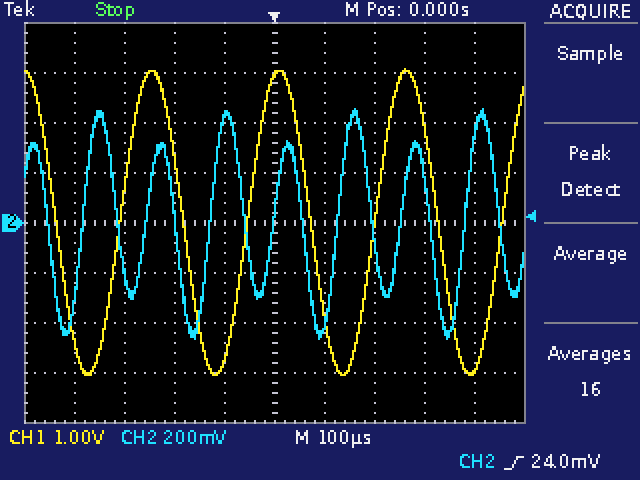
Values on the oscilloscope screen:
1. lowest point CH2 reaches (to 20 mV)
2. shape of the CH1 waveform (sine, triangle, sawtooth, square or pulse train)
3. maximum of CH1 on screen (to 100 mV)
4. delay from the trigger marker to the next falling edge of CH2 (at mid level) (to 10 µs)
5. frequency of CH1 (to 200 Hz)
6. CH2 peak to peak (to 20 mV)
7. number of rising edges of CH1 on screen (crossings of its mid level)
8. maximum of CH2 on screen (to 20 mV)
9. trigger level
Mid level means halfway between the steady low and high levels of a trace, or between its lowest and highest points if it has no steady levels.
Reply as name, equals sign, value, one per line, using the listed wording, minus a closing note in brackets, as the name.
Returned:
lowest point CH2 reaches = -460 mV
shape of the CH1 waveform = sine
maximum of CH1 on screen = 3.1 V
delay from the trigger marker to the next falling edge of CH2 (at mid level) = 60 µs
frequency of CH1 = 4.0 kHz
CH2 peak to peak = 920 mV
number of rising edges of CH1 on screen = 4
maximum of CH2 on screen = 460 mV
trigger level = 24.0 mV
